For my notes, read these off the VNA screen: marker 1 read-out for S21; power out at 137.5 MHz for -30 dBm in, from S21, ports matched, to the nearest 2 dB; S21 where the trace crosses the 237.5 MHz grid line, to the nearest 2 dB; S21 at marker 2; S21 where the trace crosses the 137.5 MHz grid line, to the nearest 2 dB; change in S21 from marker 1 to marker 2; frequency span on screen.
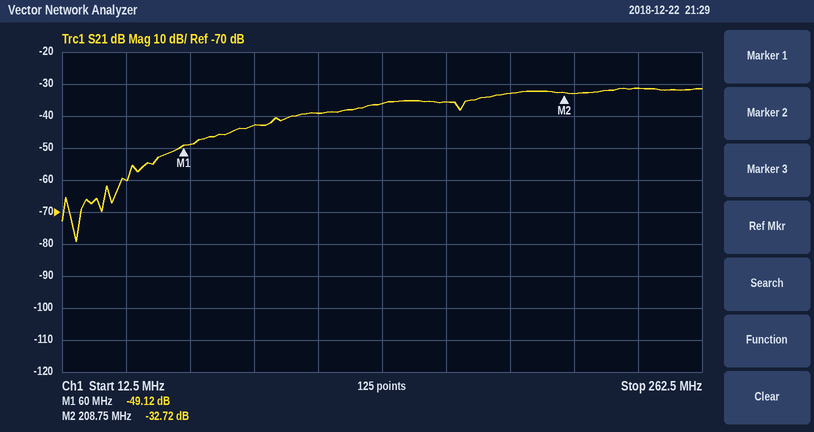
-49.12 dB
-66 dBm
-32 dB
-32.72 dB
-36 dB
16.40 dB
250 MHz
